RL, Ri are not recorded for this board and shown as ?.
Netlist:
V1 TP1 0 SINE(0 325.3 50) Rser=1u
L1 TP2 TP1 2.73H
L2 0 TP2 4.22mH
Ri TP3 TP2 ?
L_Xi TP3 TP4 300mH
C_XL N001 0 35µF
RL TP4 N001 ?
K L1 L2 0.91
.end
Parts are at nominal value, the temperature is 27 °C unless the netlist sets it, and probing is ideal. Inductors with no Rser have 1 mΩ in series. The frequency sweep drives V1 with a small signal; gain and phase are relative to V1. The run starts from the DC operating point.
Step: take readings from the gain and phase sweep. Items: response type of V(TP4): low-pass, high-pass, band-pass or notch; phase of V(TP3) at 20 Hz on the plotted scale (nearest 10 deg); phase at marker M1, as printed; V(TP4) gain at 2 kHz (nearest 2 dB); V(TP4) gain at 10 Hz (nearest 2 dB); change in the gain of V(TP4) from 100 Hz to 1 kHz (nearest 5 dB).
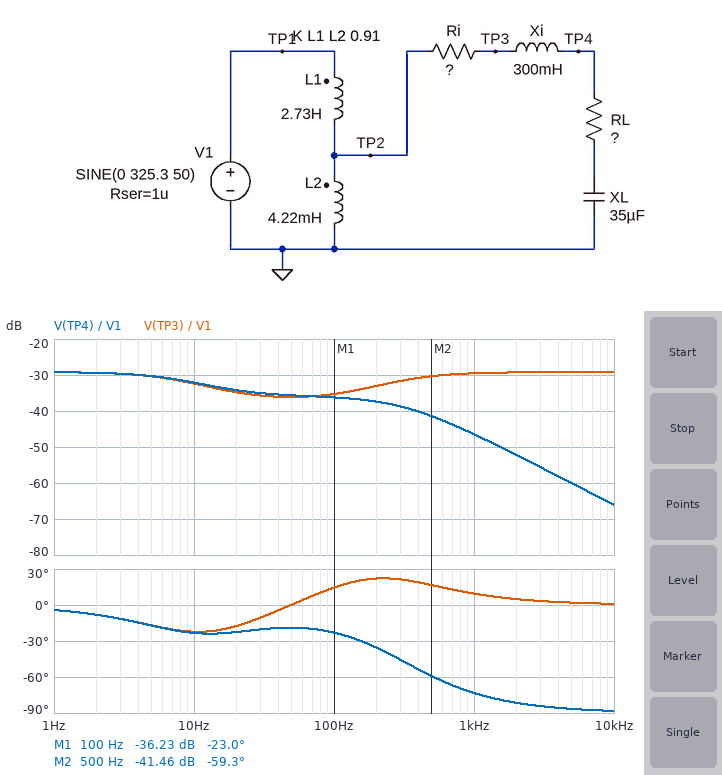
low-pass
-20 deg
-23.0 deg
-52 dB
-32 dB
-10 dB
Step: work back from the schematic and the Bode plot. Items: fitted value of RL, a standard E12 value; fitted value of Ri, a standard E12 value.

270 Ω
330 Ω
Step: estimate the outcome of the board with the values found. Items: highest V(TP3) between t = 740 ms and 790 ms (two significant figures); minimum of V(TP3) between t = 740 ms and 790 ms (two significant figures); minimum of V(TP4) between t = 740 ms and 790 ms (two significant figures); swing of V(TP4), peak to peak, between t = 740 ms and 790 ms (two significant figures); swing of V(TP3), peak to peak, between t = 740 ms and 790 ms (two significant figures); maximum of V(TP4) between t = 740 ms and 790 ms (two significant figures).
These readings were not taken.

5.1 V
-5.1 V
-5.4 V
11 V
10 V
5.4 V
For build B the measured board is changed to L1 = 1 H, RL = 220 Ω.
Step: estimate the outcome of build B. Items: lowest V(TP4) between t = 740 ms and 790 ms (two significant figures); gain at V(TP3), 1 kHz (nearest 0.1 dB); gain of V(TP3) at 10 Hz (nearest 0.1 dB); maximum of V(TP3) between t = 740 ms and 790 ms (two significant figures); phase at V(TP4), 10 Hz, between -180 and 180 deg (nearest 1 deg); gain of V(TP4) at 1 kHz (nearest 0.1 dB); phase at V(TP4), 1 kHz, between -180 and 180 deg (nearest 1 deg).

-7.9 V
-25.3 dB
-28.1 dB
7.3 V
-26 deg
-44.0 dB
-75 deg
